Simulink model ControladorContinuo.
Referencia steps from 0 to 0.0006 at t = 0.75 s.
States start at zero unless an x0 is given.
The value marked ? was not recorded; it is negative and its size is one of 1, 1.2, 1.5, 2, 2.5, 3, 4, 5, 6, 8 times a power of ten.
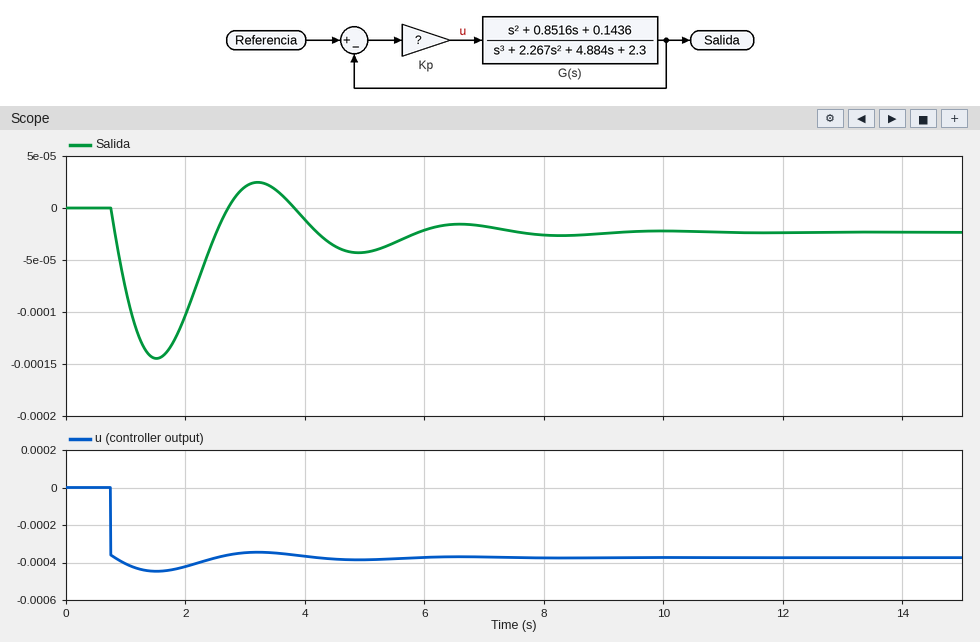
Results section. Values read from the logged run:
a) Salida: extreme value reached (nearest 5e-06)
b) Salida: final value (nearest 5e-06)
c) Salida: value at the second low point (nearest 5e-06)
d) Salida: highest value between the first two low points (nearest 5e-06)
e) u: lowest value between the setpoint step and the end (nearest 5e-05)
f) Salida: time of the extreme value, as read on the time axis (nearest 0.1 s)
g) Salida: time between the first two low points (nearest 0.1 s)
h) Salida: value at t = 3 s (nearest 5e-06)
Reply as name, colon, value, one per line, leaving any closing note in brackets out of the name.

Salida: extreme value reached: -0.000145
Salida: final value: -0.000025
Salida: value at the second low point: -0.000045
Salida: highest value between the first two low points: 0.000025
u: lowest value between the setpoint step and the end: -0.00045
Salida: time of the extreme value, as read on the time axis: 1.5 s
Salida: time between the first two low points: 3.4 s
Salida: value at t = 3 s: 0.000020
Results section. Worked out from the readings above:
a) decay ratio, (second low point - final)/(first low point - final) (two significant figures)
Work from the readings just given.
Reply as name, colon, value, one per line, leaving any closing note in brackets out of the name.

decay ratio, (second low point - final)/(first low point - final): 0.17
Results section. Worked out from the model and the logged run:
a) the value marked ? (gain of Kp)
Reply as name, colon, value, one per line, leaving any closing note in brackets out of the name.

the value marked ?: -0.6
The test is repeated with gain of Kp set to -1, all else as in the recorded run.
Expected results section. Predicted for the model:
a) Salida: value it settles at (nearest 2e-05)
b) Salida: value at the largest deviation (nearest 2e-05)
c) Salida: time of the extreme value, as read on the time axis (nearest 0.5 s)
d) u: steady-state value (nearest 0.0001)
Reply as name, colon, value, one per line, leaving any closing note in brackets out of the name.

Salida: value it settles at: -0.00004
Salida: value at the largest deviation: -0.00028
Salida: time of the extreme value, as read on the time axis: 1.5 s
u: steady-state value: -0.0006
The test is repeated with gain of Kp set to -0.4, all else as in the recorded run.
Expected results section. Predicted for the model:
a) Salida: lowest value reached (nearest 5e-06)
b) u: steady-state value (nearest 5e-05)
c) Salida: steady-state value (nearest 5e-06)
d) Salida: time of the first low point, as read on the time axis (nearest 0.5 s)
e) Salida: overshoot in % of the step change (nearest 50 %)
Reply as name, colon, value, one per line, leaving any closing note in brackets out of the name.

Salida: lowest value reached: -0.000090
u: steady-state value: -0.00025
Salida: steady-state value: -0.000015
Salida: time of the first low point, as read on the time axis: 1.5 s
Salida: overshoot in % of the step change: 500 %
